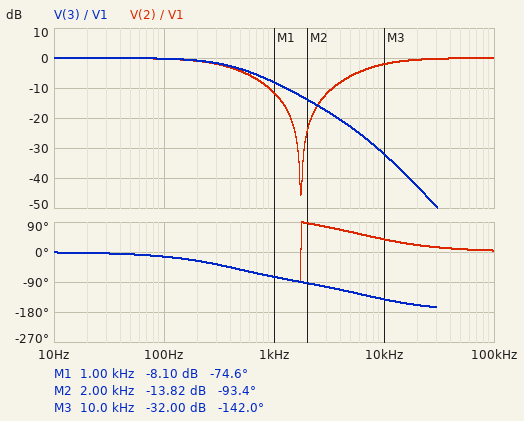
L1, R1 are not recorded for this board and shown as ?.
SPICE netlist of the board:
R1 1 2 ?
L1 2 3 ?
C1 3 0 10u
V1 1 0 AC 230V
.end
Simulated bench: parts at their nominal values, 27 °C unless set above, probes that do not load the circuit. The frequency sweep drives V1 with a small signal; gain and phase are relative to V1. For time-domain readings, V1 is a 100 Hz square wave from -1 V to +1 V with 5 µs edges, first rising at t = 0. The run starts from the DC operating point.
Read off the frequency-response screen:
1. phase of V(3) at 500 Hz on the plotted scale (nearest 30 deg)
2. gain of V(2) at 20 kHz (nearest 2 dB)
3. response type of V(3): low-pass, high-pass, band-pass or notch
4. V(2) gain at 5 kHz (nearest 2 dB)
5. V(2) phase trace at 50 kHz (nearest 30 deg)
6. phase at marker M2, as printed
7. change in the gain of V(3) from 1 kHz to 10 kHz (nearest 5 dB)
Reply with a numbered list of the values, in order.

1. -60 deg
2. 0 dB
3. low-pass
4. -6 dB
5. 0 deg
6. -93.4 deg
7. -25 dB
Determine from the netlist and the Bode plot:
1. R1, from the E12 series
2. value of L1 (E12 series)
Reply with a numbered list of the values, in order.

1. 39 Ω
2. 820 µH
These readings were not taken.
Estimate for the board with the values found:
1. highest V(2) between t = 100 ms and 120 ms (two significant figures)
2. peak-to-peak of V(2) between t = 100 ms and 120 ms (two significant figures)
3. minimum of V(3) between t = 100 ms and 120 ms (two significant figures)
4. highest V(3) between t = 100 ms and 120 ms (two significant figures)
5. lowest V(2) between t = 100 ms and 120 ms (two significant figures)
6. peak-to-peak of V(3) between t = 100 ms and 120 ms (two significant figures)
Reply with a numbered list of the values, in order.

1. 1.0 V
2. 2.0 V
3. -1.0 V
4. 1.0 V
5. -1.0 V
6. 2.0 V
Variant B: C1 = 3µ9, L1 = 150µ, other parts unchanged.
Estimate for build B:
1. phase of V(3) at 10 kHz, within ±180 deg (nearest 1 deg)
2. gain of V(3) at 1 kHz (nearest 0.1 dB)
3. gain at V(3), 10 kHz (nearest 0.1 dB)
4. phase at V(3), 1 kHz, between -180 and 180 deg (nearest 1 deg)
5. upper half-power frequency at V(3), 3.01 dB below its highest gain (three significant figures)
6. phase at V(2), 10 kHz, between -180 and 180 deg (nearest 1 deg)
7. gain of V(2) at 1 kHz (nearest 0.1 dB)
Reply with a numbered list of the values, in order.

1. -98 deg
2. -2.7 dB
3. -19.7 dB
4. -44 deg
5. 1.07 kHz
6. 82 deg
7. -2.9 dB
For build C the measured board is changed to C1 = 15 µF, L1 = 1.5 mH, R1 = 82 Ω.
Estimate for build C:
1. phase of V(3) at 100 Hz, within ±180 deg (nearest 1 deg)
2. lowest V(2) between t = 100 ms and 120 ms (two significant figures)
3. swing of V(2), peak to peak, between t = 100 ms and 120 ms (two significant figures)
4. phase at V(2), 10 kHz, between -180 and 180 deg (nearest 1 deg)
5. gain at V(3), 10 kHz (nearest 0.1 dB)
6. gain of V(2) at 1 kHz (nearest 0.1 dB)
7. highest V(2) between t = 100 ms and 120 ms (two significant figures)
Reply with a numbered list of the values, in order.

1. -38 deg
2. -970 mV
3. 1.9 V
4. 41 deg
5. -41.4 dB
6. -36.8 dB
7. 970 mV
